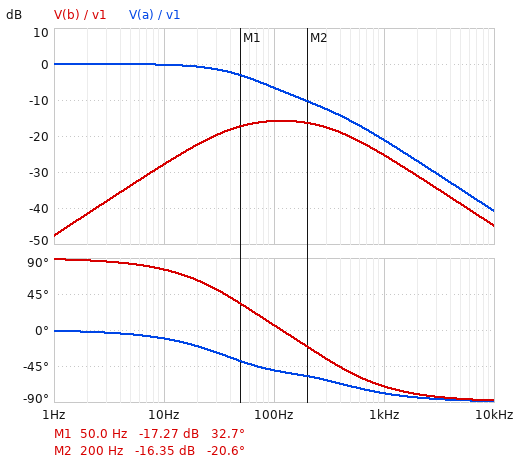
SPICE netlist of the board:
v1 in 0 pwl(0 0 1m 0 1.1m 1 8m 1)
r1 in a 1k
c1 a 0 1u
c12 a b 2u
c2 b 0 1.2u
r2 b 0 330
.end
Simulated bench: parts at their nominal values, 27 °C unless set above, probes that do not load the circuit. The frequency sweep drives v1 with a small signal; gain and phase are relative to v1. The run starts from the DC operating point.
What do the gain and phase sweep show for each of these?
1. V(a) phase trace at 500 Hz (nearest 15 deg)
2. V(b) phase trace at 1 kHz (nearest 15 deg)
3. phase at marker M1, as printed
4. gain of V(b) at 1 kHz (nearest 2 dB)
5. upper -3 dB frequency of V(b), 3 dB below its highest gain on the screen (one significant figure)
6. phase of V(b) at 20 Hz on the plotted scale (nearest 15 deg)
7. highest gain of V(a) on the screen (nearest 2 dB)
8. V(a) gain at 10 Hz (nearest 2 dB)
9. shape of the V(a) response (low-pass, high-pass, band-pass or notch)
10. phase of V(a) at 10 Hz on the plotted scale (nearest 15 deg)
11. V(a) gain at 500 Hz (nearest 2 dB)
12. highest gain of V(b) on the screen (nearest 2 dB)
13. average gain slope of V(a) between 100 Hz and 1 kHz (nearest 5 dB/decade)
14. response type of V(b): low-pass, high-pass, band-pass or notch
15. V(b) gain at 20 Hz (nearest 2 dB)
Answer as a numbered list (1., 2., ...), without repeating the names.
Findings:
1. -75 deg
2. -75 deg
3. 32.7 deg
4. -26 dB
5. 400 Hz
6. 60 deg
7. 0 dB
8. 0 dB
9. low-pass
10. -15 deg
11. -16 dB
12. -16 dB
13. -15 dB/decade
14. band-pass
15. -22 dB
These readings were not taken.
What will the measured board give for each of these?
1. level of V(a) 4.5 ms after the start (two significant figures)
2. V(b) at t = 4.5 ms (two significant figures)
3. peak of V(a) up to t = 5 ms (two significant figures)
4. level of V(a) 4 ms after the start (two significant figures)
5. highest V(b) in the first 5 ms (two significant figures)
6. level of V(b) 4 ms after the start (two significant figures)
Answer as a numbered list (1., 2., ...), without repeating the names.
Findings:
1. 690 mV
2. 82 mV
3. 730 mV
4. 640 mV
5. 130 mV
6. 94 mV
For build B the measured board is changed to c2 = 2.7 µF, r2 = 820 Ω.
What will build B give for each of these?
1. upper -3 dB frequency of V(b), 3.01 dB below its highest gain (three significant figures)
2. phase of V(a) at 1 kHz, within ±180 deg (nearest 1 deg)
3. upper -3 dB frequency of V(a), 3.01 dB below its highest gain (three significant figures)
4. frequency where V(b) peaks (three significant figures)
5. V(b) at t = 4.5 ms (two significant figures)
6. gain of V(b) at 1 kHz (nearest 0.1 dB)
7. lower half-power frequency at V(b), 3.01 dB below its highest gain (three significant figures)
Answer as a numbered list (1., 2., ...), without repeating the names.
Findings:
1. 152 Hz
2. -85 deg
3. 54.1 Hz
4. 55.3 Hz
5. 180 mV
6. -30.1 dB
7. 20.1 Hz
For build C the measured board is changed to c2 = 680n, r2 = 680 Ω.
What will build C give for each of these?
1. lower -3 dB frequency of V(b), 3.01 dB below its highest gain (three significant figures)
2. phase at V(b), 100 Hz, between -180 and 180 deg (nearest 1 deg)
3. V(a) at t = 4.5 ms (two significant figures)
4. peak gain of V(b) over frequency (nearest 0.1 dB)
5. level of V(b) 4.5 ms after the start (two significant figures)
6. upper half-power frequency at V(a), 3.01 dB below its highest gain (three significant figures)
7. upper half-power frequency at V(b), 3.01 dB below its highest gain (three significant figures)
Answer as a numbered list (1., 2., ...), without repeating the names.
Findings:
1. 29.8 Hz
2. -2 deg
3. 710 mV
4. -11.0 dB
5. 170 mV
6. 46.4 Hz
7. 309 Hz
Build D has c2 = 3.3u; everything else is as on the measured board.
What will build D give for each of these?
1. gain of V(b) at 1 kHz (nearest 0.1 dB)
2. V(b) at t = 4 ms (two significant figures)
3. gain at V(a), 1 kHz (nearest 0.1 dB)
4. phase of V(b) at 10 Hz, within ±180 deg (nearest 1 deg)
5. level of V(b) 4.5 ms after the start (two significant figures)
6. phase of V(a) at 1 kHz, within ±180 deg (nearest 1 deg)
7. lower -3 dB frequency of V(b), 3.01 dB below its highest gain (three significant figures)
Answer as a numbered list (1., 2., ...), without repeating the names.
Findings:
1. -31.6 dB
2. 97 mV
3. -23.1 dB
4. 73 deg
5. 89 mV
6. -84 deg
7. 29.1 Hz
